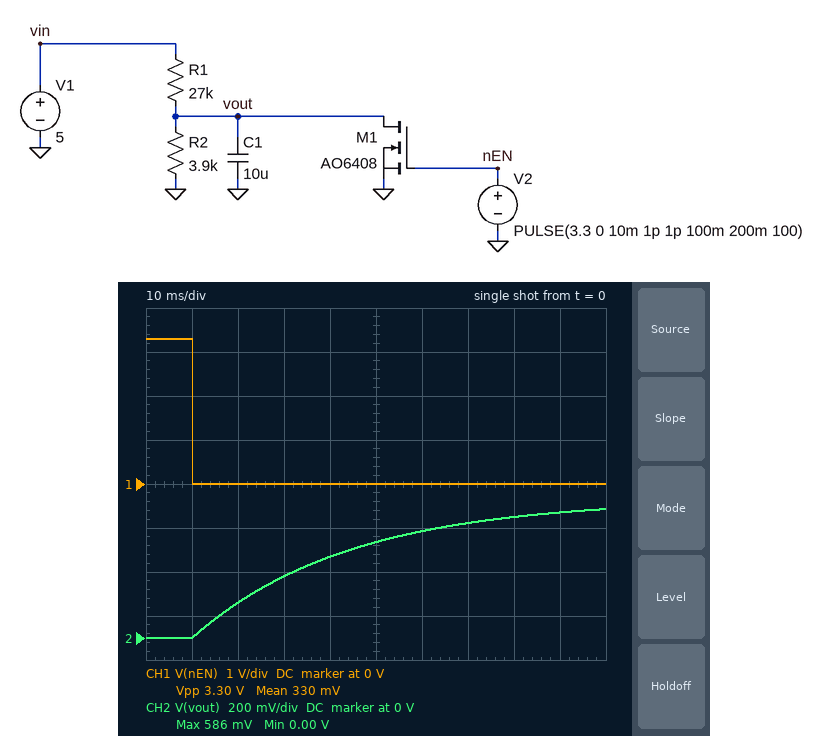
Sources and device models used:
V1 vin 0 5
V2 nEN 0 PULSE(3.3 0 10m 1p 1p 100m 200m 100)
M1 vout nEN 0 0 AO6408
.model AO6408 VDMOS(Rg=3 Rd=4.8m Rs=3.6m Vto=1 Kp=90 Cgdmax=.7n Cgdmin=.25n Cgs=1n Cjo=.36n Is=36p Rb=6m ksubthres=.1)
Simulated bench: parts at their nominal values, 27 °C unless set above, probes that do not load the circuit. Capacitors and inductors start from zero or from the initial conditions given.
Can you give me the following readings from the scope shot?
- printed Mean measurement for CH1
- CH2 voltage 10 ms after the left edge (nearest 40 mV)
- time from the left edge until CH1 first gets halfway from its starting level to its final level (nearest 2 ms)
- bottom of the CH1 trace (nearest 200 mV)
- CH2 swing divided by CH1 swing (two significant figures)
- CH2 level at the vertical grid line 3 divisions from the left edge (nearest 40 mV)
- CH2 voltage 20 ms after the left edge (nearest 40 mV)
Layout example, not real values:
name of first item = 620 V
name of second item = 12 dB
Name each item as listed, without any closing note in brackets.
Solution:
printed Mean measurement for CH1 = 330 mV
CH2 voltage 10 ms after the left edge = 0 V
time from the left edge until CH1 first gets halfway from its starting level to its final level = 10 ms
bottom of the CH1 trace = 0 V
CH2 swing divided by CH1 swing = 0.18
CH2 level at the vertical grid line 3 divisions from the left edge = 280 mV
CH2 voltage 20 ms after the left edge = 160 mV
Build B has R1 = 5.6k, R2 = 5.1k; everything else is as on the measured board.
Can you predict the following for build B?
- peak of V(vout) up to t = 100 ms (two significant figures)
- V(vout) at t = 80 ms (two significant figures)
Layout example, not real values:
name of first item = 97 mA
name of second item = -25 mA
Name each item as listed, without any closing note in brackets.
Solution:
peak of V(vout) up to t = 100 ms = 2.3 V
V(vout) at t = 80 ms = 2.2 V
